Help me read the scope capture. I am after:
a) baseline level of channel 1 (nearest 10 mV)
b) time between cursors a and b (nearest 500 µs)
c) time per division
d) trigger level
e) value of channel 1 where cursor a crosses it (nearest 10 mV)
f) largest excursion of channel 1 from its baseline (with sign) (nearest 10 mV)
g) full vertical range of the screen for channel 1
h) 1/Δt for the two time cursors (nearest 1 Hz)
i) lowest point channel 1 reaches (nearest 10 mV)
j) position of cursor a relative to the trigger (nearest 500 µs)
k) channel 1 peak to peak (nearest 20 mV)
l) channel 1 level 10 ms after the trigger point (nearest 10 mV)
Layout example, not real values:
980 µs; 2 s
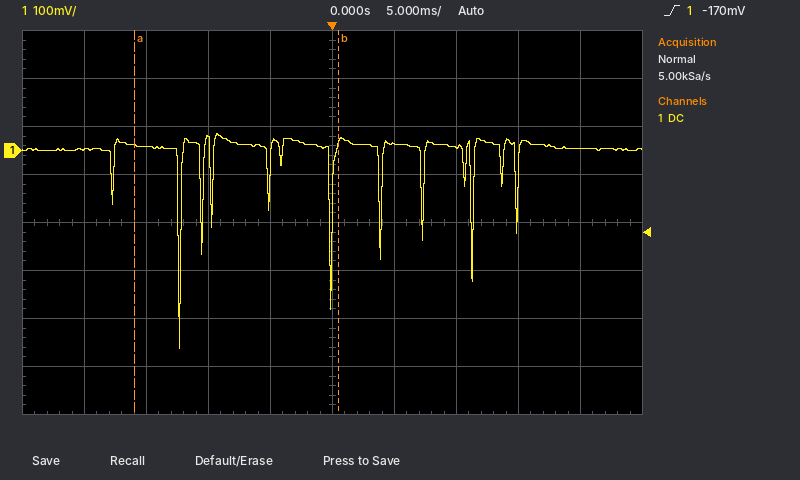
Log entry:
10 mV; 16.5 ms; 5 ms; -170 mV; 10 mV; -420 mV; 800 mV; 61 Hz; -410 mV; -16.0 ms; 440 mV; 10 mV
